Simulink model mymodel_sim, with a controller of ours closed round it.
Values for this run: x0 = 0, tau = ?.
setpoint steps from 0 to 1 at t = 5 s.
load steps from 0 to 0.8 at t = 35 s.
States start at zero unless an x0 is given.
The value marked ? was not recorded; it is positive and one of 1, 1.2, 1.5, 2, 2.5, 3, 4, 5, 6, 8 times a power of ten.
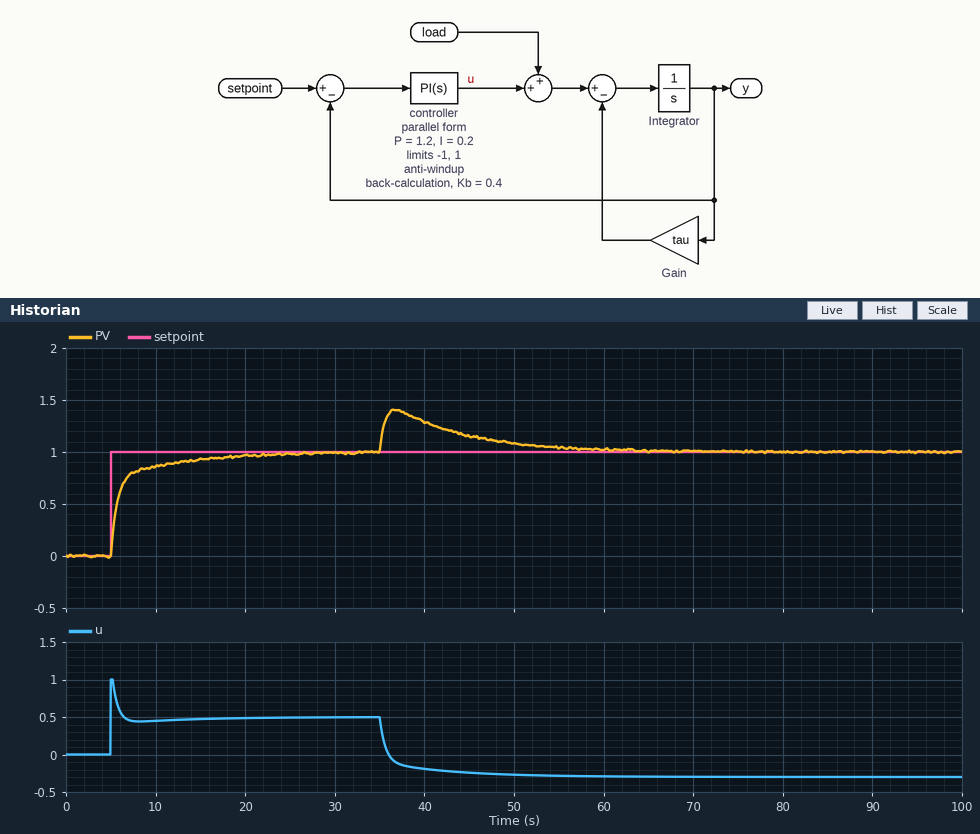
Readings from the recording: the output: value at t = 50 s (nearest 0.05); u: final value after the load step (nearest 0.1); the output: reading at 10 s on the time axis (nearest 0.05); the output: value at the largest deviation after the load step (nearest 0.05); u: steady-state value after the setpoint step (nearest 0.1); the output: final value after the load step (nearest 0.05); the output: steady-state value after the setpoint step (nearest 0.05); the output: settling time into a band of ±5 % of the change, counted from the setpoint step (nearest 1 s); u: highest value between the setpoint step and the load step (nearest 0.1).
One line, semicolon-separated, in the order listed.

1.10; -0.3; 0.85; 1.40; 0.5; 1.00; 1.00; 13 s; 1.0
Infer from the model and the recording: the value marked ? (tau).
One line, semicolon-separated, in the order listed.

0.5
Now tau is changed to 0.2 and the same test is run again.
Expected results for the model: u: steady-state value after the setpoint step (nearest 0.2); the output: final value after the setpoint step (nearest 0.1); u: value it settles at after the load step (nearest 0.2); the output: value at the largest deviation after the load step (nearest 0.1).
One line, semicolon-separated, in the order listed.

0.2; 1.0; -0.6; 1.5
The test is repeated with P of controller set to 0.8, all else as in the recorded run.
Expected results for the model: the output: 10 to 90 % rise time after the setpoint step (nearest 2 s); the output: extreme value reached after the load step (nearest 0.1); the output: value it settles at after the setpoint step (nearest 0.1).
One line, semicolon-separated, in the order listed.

6 s; 1.5; 1.0
